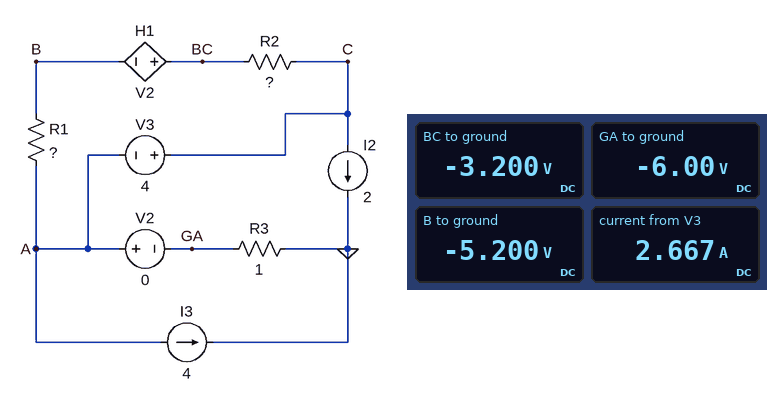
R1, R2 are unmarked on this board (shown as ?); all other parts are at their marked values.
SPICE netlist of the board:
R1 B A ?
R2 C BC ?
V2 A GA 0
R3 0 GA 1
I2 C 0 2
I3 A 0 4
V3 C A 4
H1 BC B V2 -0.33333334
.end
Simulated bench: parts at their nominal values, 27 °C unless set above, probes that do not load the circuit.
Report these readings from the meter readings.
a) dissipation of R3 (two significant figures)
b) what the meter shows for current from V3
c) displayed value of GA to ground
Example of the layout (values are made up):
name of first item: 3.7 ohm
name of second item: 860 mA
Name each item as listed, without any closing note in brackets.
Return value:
dissipation of R3: 36 W
what the meter shows for current from V3: 2.667 A
displayed value of GA to ground: -6.00 V
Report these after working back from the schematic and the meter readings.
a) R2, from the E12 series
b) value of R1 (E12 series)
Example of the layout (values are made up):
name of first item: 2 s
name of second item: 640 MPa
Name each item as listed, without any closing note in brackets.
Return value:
R2, from the E12 series: 1.8 Ω
value of R1: 1.2 Ω
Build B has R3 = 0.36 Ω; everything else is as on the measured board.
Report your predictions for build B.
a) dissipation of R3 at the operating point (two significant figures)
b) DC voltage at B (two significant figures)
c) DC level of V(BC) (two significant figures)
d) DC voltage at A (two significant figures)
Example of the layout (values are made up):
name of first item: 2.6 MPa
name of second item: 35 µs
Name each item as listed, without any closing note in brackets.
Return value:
dissipation of R3 at the operating point: 13 W
DC voltage at B: -1.4 V
DC level of V(BC): 640 mV
DC voltage at A: -2.2 V
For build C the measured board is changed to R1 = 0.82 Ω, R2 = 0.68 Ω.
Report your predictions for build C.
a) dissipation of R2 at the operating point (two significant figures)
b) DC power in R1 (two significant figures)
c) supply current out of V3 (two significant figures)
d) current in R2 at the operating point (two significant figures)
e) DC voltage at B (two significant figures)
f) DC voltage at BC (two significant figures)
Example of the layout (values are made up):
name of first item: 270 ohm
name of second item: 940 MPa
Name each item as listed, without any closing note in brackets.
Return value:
dissipation of R2 at the operating point: 1.2 W
DC power in R1: 1.5 W
supply current out of V3: 3.3 A
current in R2 at the operating point: 1.3 A
DC voltage at B: -4.9 V
DC voltage at BC: -2.9 V
